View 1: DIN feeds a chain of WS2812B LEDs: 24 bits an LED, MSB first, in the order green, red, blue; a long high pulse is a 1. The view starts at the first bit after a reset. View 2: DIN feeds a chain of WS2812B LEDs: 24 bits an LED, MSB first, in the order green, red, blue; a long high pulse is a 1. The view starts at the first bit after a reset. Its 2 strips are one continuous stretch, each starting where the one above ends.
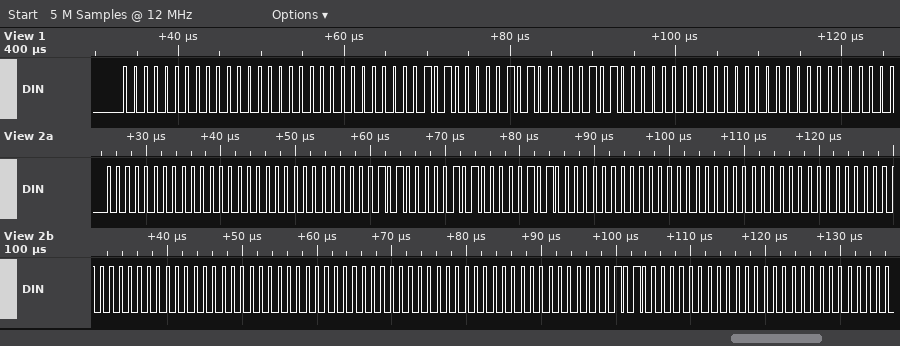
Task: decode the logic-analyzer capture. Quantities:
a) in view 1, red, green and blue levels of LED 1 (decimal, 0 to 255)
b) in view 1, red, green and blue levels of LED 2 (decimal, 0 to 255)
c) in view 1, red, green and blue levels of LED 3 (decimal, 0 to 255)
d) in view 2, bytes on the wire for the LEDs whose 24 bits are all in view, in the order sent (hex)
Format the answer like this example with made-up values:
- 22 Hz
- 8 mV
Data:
- 0, 0, 0
- 5, 5, 5
- 0, 0, 0
- 00 00 00 05 05 05 00 00 00 00 00 00 00 00 00 00 00 0A 00 00 00
